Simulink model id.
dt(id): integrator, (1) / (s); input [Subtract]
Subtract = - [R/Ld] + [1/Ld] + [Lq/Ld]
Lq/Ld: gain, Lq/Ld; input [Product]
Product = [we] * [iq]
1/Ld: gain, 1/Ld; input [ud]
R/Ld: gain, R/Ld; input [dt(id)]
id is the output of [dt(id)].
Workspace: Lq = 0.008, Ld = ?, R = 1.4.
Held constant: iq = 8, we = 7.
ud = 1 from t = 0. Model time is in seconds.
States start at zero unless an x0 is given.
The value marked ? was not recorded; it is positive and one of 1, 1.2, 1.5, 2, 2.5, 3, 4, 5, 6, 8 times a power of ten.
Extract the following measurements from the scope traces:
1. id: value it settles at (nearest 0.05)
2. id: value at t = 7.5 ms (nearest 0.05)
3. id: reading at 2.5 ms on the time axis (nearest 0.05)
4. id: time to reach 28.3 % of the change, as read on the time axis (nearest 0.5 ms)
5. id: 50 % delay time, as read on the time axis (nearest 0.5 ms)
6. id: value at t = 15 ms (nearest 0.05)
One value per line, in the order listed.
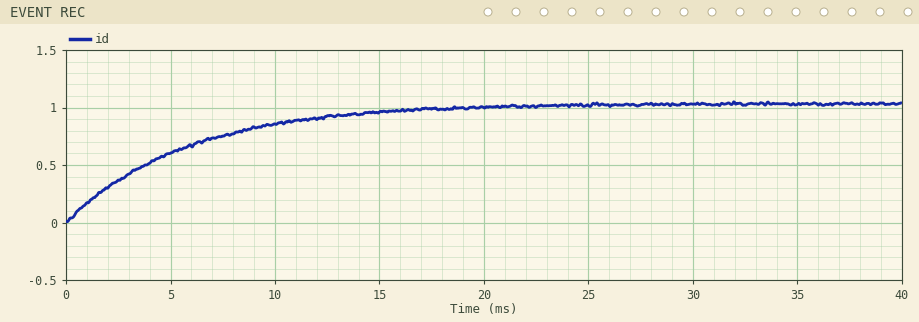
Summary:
1.05
0.75
0.35
2.0 ms
4.0 ms
0.95
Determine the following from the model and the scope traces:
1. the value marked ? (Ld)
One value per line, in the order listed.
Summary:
0.008
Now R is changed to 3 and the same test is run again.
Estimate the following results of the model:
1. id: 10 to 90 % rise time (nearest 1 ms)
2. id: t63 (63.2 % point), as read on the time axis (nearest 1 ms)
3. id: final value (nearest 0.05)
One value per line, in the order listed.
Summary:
6 ms
3 ms
0.50
